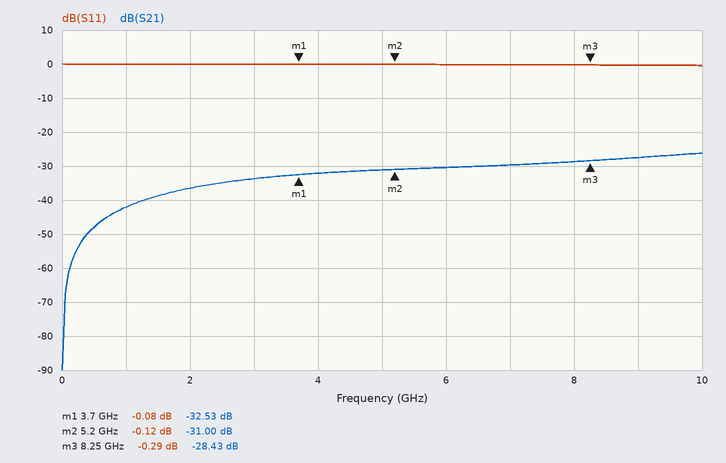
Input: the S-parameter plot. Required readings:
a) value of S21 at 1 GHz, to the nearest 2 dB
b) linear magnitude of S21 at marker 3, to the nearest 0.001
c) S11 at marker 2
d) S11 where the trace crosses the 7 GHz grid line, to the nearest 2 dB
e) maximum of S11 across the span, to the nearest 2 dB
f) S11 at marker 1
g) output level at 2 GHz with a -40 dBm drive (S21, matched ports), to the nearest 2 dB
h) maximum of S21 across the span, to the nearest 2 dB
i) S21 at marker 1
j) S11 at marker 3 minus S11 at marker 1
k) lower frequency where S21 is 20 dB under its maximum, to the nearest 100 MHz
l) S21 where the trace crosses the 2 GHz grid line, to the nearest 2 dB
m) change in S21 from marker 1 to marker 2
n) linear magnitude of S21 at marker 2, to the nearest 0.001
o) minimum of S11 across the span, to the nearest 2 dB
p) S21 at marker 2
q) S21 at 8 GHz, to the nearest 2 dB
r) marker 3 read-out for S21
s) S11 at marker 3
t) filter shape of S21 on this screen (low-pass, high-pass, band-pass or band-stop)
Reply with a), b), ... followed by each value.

a) -42 dB
b) 0.038
c) -0.12 dB
d) 0 dB
e) 0 dB
f) -0.08 dB
g) -76 dBm
h) -26 dB
i) -32.53 dB
j) -0.21 dB
k) 600 MHz
l) -36 dB
m) 1.53 dB
n) 0.028
o) 0 dB
p) -31.00 dB
q) -28 dB
r) -28.43 dB
s) -0.29 dB
t) high-pass
